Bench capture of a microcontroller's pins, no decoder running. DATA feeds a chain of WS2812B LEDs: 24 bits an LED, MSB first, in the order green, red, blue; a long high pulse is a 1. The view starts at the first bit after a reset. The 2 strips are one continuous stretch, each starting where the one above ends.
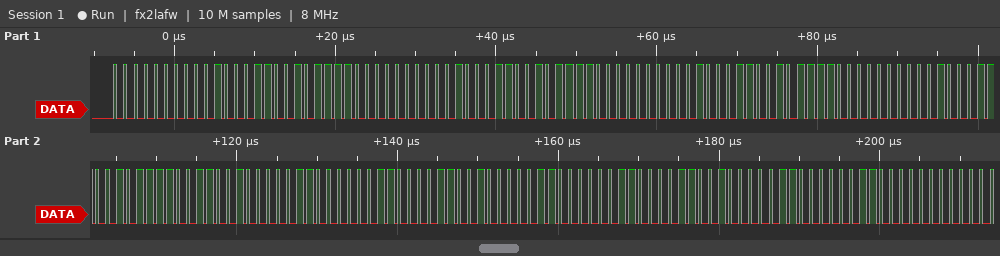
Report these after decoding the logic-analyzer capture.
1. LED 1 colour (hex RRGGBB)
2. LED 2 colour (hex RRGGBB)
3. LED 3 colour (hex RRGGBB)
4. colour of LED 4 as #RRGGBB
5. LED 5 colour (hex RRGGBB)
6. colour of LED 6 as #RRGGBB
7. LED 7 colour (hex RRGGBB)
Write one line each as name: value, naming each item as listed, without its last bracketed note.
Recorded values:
LED 1 colour: #23002F
LED 2 colour: #23002F
LED 3 colour: #23002F
colour of LED 4 as #RRGGBB: #23002F
LED 5 colour: #0C320C
colour of LED 6 as #RRGGBB: #0C320C
LED 7 colour: #0C320C
